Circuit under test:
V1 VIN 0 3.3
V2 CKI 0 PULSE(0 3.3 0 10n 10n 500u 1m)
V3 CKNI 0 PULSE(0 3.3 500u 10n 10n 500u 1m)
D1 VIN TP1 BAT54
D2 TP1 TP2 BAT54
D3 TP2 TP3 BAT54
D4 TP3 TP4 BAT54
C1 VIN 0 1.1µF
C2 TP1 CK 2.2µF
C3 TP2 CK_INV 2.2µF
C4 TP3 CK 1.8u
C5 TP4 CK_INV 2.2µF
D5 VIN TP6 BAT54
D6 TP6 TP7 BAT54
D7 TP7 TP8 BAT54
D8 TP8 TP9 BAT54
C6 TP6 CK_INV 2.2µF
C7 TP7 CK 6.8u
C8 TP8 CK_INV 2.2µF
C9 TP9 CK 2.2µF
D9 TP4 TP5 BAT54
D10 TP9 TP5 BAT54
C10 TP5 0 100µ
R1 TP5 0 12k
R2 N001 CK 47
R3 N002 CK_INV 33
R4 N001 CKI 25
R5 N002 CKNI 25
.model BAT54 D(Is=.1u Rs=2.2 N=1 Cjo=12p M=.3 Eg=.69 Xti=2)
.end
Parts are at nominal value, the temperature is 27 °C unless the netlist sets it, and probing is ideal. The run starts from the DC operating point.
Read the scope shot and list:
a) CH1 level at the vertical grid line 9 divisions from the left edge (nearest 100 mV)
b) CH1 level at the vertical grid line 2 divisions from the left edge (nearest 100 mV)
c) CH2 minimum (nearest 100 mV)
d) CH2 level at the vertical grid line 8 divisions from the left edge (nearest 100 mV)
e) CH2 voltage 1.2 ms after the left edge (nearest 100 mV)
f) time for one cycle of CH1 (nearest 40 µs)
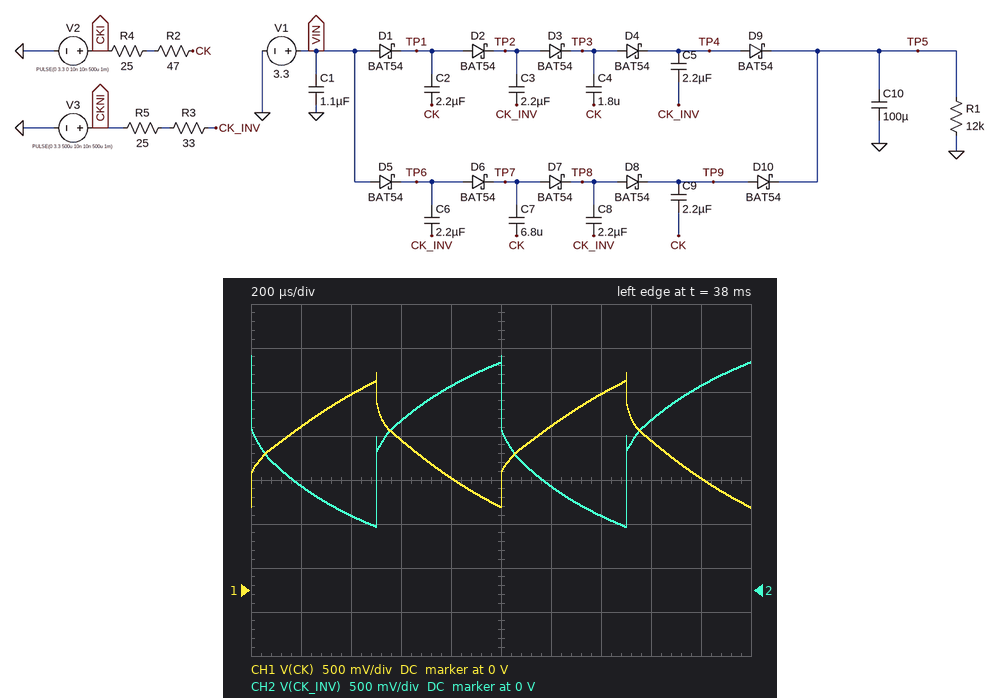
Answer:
1.3 V
2.2 V
700 mV
1.9 V
1.2 V
1.00 ms
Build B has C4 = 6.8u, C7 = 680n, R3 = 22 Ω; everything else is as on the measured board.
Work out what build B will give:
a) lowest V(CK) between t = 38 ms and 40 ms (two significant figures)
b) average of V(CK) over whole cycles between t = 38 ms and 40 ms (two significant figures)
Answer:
840 mV
1.7 V
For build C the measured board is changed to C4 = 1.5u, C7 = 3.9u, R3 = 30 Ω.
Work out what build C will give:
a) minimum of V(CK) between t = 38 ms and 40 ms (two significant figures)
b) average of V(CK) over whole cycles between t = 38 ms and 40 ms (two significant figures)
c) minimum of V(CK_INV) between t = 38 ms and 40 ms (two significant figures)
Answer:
910 mV
1.7 V
650 mV
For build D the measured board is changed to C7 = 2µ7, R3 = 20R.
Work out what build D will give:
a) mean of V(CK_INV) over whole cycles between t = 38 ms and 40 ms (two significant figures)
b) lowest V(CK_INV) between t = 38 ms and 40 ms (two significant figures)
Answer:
1.7 V
520 mV
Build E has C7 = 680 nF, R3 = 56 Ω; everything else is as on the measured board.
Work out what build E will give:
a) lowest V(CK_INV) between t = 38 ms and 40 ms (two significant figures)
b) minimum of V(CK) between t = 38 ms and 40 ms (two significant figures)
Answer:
840 mV
720 mV
